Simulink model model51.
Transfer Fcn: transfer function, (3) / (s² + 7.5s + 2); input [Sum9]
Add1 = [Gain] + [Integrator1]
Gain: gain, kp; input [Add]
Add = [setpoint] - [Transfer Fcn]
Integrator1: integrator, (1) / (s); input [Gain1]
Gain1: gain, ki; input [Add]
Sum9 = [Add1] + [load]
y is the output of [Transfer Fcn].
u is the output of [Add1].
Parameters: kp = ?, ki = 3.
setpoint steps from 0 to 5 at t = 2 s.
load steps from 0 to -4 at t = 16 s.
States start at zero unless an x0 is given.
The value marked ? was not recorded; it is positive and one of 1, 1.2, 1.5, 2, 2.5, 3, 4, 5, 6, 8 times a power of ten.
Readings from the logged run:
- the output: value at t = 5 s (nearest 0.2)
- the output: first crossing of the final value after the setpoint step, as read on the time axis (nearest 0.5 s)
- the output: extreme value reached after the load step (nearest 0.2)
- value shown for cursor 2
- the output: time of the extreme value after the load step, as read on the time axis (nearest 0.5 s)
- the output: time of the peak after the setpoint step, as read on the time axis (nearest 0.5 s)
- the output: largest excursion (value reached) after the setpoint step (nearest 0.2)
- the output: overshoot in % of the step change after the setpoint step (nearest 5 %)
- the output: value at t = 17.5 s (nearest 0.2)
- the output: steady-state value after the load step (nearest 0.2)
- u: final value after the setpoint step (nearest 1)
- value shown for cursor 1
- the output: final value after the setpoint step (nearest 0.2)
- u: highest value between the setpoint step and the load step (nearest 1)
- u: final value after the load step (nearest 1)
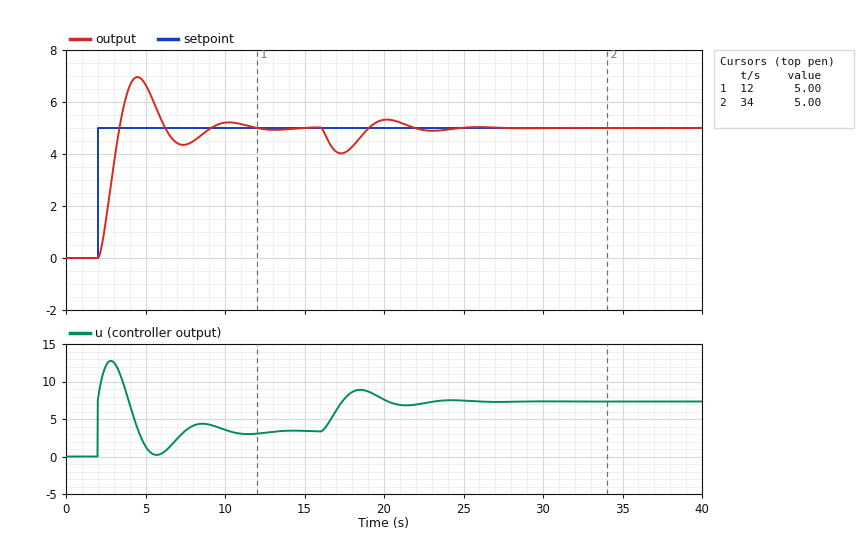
6.6
3.5 s
4.0
5.00
17.5 s
4.5 s
7.0
40 %
4.0
5.0
3
5.00
5.0
13
7
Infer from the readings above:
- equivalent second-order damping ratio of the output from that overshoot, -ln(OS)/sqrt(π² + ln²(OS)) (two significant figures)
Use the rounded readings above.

0.28
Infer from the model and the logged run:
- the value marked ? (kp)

1.5
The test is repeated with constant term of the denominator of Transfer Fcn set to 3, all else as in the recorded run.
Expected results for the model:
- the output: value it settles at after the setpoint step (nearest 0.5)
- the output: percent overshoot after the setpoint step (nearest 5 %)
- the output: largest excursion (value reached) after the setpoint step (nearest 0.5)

5.0
30 %
6.5
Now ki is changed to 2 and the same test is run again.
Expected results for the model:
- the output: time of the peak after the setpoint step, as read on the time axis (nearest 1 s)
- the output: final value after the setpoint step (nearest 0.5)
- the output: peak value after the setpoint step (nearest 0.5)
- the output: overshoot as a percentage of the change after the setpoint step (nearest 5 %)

5 s
5.0
6.5
30 %
